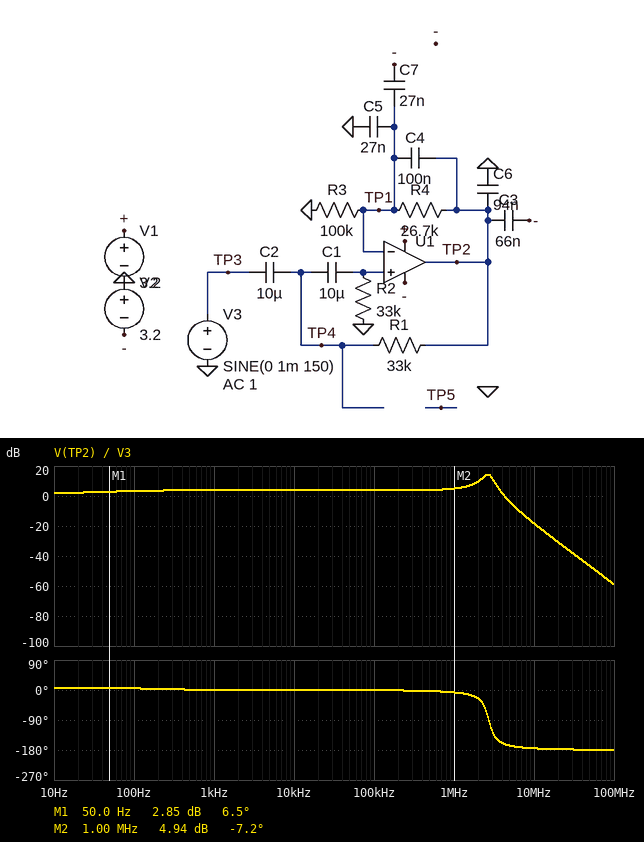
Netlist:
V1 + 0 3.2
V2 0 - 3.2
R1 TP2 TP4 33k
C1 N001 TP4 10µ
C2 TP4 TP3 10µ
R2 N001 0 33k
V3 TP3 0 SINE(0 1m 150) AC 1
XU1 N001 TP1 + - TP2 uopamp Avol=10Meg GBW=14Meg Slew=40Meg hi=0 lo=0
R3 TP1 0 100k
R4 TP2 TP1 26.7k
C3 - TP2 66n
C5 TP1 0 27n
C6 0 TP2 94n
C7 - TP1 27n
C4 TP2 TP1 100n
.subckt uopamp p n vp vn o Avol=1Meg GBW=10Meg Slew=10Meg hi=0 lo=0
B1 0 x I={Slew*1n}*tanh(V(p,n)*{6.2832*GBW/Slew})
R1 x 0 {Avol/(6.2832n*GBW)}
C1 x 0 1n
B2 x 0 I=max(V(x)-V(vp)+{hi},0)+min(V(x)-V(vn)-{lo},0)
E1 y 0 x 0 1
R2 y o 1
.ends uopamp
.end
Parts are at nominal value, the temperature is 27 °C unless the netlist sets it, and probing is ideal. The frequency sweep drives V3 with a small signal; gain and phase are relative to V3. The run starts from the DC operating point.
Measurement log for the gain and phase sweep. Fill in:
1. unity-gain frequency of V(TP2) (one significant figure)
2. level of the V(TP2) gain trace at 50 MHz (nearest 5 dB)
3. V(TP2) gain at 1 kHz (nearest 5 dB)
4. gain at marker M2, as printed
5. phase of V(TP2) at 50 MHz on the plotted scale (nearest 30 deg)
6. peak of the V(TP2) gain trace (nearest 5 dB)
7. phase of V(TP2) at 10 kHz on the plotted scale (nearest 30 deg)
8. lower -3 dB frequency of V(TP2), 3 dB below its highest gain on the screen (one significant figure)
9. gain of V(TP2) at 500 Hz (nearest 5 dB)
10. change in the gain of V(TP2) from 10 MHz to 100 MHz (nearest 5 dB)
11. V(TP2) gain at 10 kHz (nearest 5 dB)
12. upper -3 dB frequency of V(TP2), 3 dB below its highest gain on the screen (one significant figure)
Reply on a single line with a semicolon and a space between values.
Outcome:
4 MHz; -45 dB; 5 dB; 4.94 dB; -180 deg; 15 dB; 0 deg; 2 MHz; 5 dB; -40 dB; 5 dB; 3 MHz
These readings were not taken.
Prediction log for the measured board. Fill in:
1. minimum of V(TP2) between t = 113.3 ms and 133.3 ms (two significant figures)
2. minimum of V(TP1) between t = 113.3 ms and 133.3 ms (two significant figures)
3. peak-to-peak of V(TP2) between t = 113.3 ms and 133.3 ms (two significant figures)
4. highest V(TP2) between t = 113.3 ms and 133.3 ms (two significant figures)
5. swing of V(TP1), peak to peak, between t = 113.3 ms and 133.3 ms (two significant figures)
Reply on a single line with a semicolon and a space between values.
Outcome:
-1.5 mV; -1.0 mV; 3.0 mV; 1.5 mV; 2.0 mV
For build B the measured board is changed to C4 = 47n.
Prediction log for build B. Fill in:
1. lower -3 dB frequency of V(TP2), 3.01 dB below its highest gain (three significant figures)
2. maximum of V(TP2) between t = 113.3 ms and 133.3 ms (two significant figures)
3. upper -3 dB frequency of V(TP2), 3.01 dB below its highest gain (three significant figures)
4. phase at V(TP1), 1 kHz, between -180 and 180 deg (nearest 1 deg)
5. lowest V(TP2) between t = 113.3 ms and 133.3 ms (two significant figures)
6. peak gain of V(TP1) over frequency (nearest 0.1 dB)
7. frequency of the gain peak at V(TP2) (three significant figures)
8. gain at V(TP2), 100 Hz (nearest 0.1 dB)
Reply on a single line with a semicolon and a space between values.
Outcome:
1.80 MHz; 1.8 mV; 2.69 MHz; 0 deg; -1.8 mV; 8.9 dB; 2.29 MHz; 4.4 dB
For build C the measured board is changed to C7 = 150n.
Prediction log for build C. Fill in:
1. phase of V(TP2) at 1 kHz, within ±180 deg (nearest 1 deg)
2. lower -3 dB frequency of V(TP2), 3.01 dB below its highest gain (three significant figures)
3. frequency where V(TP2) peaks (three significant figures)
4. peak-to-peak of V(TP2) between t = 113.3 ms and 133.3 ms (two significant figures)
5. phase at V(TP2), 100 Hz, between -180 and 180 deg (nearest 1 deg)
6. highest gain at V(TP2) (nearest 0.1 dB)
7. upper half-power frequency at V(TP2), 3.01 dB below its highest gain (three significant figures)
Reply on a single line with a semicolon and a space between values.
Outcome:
2 deg; 1.42 MHz; 1.83 MHz; 5.2 mV; 16 deg; 17.5 dB; 2.16 MHz
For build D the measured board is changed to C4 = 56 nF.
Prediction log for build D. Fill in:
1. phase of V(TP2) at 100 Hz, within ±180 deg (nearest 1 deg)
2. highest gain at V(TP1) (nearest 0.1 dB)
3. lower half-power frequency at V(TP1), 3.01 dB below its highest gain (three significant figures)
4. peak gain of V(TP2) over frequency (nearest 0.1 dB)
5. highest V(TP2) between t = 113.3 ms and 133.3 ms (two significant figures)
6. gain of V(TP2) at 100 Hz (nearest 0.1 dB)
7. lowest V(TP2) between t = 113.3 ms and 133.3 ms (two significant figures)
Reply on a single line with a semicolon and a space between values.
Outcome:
13 deg; 9.4 dB; 1.91 MHz; 15.2 dB; 1.8 mV; 4.3 dB; -1.8 mV
